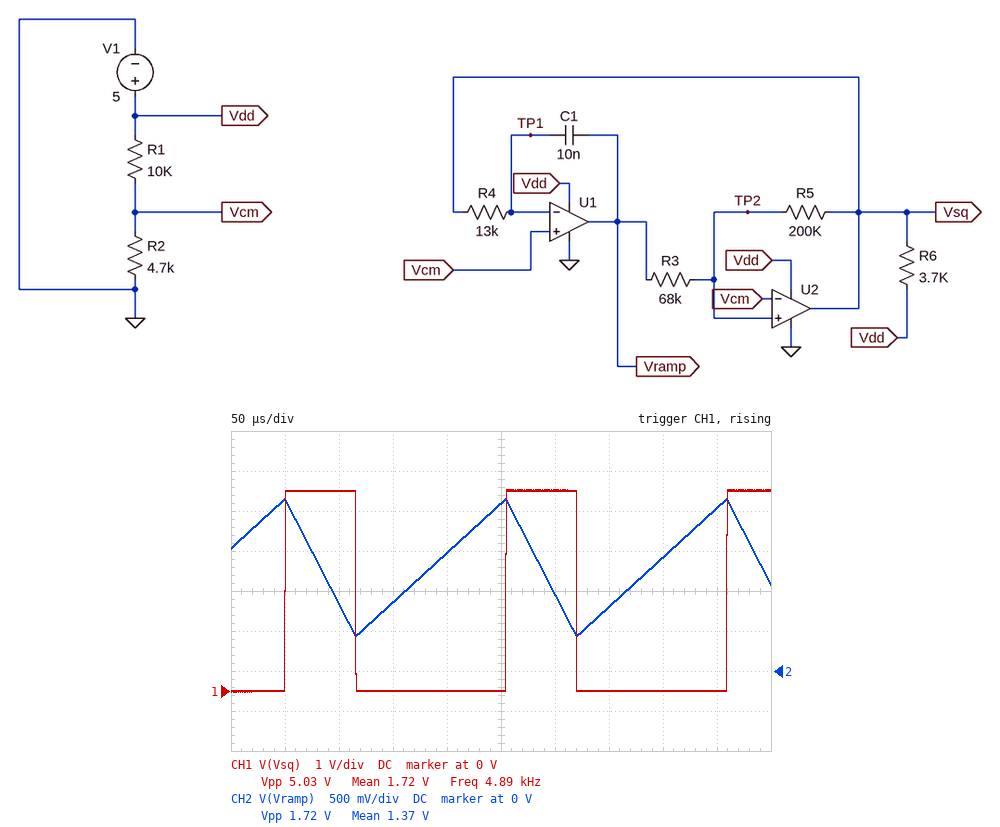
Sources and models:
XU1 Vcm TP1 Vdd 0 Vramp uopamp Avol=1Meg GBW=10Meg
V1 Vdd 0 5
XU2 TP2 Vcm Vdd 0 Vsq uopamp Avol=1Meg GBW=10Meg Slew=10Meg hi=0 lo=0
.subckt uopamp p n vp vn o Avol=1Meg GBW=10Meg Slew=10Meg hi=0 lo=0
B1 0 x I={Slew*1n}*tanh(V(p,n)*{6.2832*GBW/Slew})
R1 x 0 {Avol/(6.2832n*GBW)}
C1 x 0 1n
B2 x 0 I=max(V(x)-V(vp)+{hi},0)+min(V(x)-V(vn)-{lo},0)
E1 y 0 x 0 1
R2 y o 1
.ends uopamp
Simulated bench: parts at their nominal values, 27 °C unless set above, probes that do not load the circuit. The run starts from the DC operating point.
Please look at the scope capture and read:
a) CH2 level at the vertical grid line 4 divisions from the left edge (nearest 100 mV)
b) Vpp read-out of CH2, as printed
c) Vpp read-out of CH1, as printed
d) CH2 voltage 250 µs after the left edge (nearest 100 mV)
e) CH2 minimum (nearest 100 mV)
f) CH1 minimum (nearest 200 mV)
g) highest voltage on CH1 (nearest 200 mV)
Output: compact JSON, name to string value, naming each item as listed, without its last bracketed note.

{"CH2 level at the vertical grid line 4 divisions from the left edge": "1.5 V", "Vpp read-out of CH2, as printed": "1.72 V", "Vpp read-out of CH1, as printed": "5.03 V", "CH2 voltage 250 µs after the left edge": "2.1 V", "CH2 minimum": "400 mV", "CH1 minimum": "0 V", "highest voltage on CH1": "5.0 V"}
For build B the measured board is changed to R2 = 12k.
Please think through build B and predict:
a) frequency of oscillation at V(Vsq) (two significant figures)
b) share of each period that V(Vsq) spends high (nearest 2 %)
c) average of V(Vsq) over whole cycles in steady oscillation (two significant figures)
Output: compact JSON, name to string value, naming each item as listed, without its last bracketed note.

{"frequency of oscillation at V(Vsq)": "5.6 kHz", "share of each period that V(Vsq) spends high": "54 %", "average of V(Vsq) over whole cycles in steady oscillation": "2.7 V"}
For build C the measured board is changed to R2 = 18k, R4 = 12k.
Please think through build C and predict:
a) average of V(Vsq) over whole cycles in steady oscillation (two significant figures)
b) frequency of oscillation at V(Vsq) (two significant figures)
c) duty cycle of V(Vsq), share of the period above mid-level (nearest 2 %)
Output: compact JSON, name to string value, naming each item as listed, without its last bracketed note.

{"average of V(Vsq) over whole cycles in steady oscillation": "3.2 V", "frequency of oscillation at V(Vsq)": "5.6 kHz", "duty cycle of V(Vsq), share of the period above mid-level": "64 %"}
